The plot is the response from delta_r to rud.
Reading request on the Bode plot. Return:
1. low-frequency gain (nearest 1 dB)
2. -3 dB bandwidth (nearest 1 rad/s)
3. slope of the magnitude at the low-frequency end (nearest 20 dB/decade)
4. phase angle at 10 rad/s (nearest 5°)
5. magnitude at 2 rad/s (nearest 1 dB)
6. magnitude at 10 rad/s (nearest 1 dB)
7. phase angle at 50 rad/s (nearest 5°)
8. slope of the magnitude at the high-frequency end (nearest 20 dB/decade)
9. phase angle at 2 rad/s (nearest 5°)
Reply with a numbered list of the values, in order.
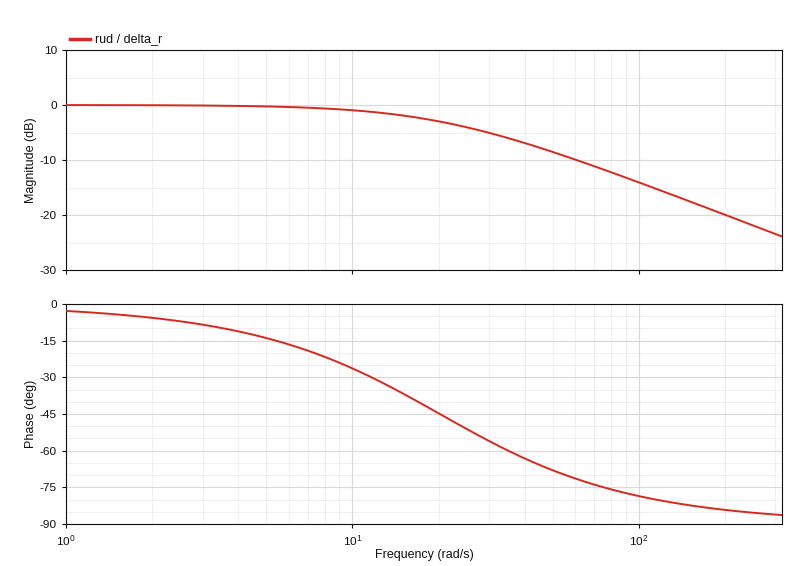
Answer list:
1. 0 dB
2. 20 rad/s
3. 0 dB/decade
4. -25°
5. 0 dB
6. -1 dB
7. -70°
8. -20 dB/decade
9. -5°
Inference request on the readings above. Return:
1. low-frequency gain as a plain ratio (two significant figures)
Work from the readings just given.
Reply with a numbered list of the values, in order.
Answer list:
1. 1.0
